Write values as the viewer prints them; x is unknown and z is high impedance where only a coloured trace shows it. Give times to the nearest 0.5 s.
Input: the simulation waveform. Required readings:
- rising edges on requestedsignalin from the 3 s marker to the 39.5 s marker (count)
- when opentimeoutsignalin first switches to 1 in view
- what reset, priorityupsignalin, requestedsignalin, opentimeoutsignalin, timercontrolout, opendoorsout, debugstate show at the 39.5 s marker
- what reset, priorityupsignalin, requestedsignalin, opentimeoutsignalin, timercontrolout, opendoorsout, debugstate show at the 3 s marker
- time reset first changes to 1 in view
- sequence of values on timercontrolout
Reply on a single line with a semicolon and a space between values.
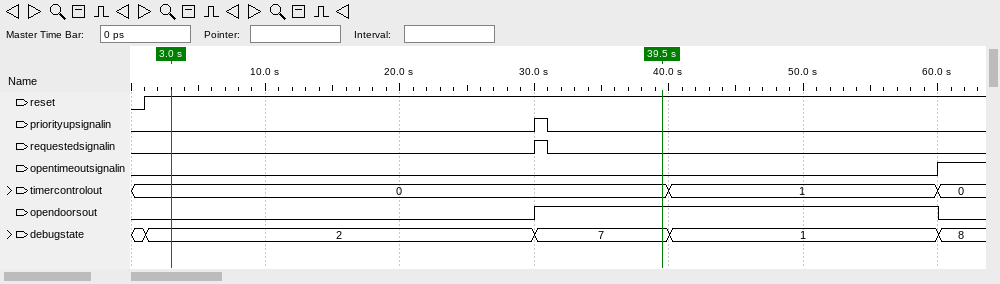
1; 60 s; reset=1, priorityupsignalin=0, requestedsignalin=0, opentimeoutsignalin=0, timercontrolout=0, opendoorsout=1, debugstate=7; reset=1, priorityupsignalin=0, requestedsignalin=0, opentimeoutsignalin=0, timercontrolout=0, opendoorsout=0, debugstate=2; 1 s; 0, 1, 0
